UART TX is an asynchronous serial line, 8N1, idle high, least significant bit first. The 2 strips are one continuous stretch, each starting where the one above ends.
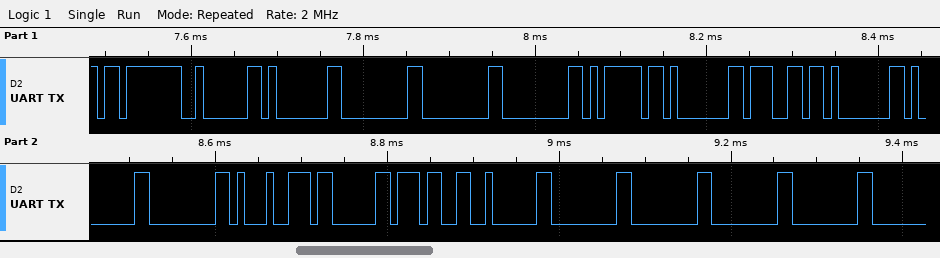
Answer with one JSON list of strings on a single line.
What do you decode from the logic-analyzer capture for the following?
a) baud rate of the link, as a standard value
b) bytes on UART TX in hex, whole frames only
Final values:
["115200 baud", "FB 02 01 00 00 00 7D 01 67 01 01 00 91 03 37 02 00 00 00 00"]
